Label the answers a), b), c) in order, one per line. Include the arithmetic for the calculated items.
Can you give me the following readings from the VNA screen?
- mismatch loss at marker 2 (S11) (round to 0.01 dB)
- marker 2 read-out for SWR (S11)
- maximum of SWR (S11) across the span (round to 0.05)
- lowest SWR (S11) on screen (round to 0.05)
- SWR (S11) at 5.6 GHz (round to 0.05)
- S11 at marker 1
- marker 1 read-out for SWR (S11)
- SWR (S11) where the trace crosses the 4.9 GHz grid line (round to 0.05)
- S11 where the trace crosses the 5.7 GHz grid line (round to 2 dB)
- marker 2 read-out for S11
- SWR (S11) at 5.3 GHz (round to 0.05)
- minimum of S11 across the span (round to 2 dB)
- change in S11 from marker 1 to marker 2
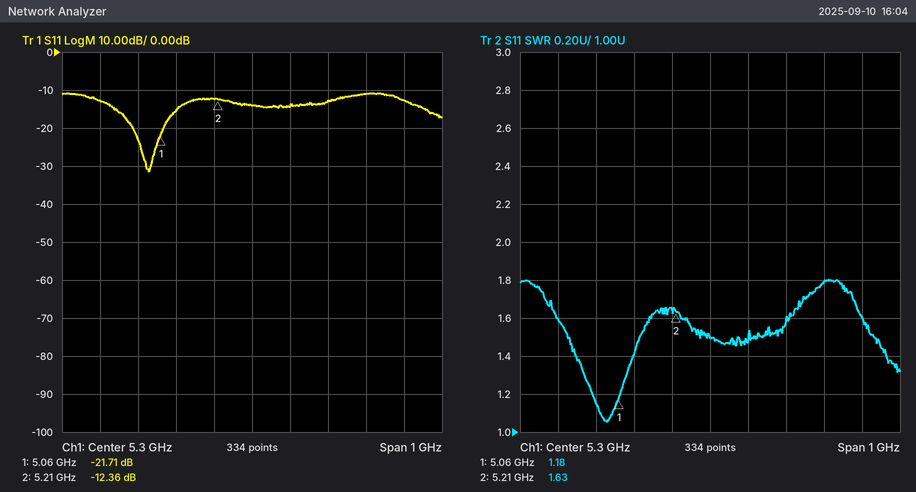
a) −10 log10(1 − 10^(-12.36/10)) ≈ 0.26 dB
b) 1.63
c) 1.80
d) 1.05
e) 1.80
f) -21.71 dB
g) 1.18
h) 1.60
i) -12 dB
j) -12.36 dB
k) 1.50
l) -32 dB
m) -12.36 − (-21.71) = 9.35 dB
